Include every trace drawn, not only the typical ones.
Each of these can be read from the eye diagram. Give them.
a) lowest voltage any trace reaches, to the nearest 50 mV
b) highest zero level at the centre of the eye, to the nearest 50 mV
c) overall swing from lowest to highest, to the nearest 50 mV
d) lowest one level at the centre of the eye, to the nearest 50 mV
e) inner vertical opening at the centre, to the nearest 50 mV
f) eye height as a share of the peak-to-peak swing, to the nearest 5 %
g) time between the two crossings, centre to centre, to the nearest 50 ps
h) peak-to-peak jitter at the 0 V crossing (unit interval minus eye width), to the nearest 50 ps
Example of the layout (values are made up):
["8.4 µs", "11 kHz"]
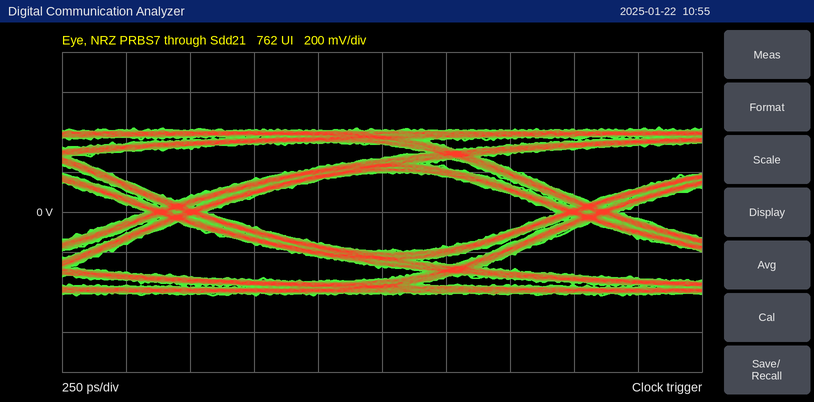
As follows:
["-400 mV", "-200 mV", "850 mV", "200 mV", "400 mV", "45 %", "1.60 ns", "250 ps"]
